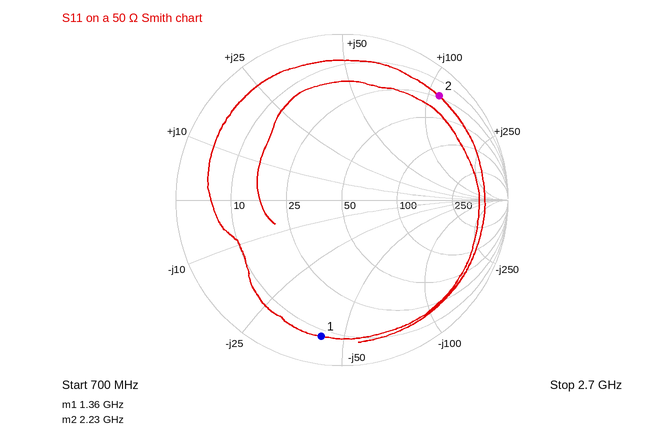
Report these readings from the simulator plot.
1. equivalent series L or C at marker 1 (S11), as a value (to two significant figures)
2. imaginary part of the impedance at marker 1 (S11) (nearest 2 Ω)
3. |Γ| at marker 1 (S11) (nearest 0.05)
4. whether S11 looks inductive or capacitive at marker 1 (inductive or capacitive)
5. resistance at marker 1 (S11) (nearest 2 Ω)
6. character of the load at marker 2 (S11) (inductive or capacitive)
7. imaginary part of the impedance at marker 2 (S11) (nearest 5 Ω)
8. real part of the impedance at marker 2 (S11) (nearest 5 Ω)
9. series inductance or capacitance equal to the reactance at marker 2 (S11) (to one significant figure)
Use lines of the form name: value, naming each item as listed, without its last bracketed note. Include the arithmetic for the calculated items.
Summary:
equivalent series L or C at marker 1 (S11), as a value: C = 1/(2π × 1.36 GHz × 42 Ω) ≈ 2.8 pF
imaginary part of the impedance at marker 1 (S11): -42 Ω
|Γ| at marker 1 (S11): 0.85
whether S11 looks inductive or capacitive at marker 1: capacitive
resistance at marker 1 (S11): 8 Ω
character of the load at marker 2 (S11): inductive
imaginary part of the impedance at marker 2 (S11): +110 Ω
real part of the impedance at marker 2 (S11): 25 Ω
series inductance or capacitance equal to the reactance at marker 2 (S11): L = 110 Ω/(2π × 2.23 GHz) ≈ 8 nH
